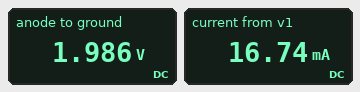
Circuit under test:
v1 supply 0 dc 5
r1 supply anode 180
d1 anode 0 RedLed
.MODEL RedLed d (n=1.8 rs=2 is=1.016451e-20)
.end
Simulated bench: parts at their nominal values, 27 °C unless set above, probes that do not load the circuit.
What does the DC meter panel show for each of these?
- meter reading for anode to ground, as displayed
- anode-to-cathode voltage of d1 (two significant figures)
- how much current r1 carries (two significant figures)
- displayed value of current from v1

1.986 V
2.0 V
17 mA
16.74 mA
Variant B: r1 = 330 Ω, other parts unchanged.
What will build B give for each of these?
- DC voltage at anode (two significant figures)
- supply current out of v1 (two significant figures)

1.9 V
9.3 mA
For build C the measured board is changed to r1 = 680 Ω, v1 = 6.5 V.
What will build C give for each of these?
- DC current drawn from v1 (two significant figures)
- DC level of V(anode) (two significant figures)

6.7 mA
1.9 V
